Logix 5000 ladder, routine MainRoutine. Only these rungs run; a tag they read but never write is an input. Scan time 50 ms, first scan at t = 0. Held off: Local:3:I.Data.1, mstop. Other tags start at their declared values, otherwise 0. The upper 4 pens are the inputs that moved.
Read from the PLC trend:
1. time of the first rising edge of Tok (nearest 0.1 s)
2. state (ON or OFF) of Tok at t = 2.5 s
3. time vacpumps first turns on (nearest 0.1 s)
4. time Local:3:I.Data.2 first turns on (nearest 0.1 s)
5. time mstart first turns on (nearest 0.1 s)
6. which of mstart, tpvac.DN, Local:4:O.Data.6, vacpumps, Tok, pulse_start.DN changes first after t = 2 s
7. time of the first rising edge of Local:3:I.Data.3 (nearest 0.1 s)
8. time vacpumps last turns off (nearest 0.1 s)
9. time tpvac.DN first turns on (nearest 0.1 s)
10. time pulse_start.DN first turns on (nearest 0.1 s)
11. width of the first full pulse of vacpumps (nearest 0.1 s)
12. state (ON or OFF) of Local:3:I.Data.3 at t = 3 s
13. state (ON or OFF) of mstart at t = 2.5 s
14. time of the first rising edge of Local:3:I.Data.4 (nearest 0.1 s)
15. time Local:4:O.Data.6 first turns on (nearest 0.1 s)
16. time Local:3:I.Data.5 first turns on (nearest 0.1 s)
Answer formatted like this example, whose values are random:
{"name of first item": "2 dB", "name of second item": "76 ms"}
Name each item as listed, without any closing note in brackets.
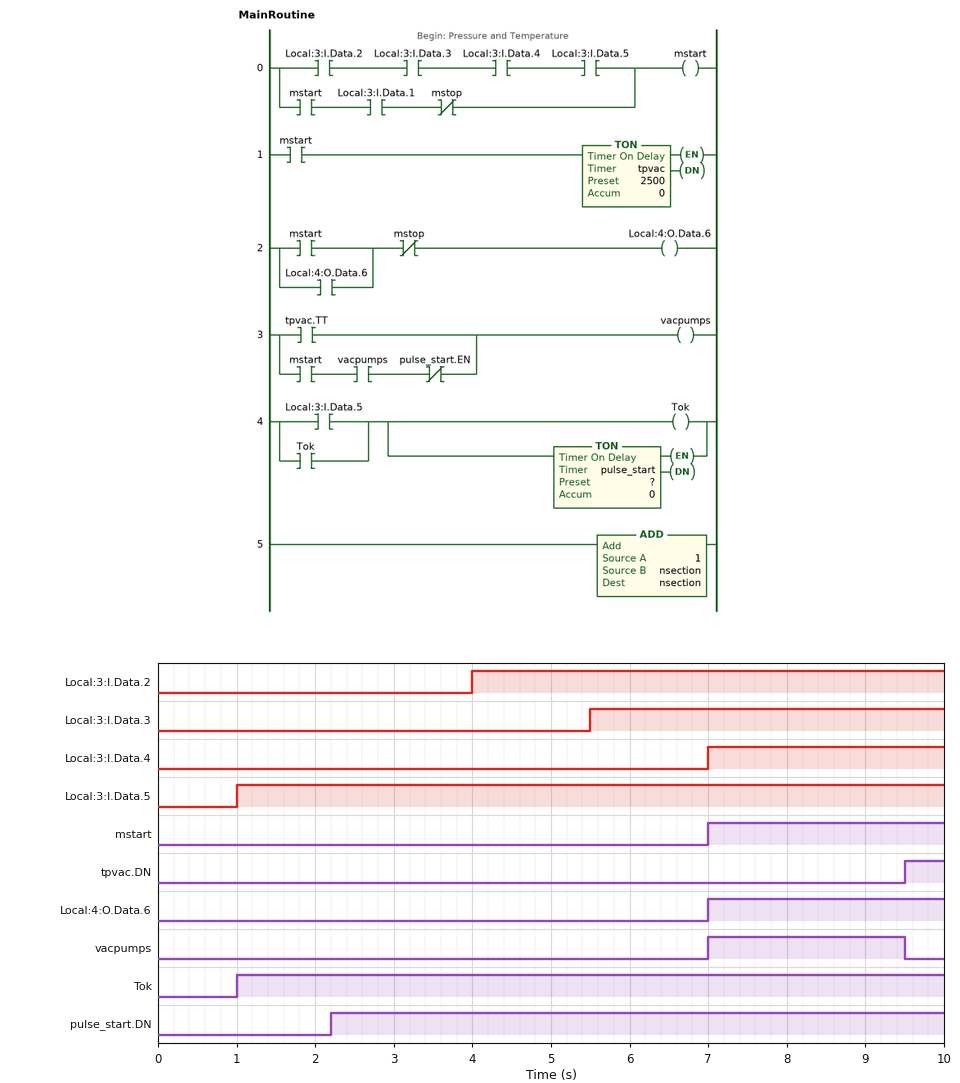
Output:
{"time of the first rising edge of Tok": "1.0 s", "state (ON or OFF) of Tok at t = 2.5 s": "ON", "time vacpumps first turns on": "7.0 s", "time Local:3:I.Data.2 first turns on": "4.0 s", "time mstart first turns on": "7.0 s", "which of mstart, tpvac.DN, Local:4:O.Data.6, vacpumps, Tok, pulse_start.DN changes first after t = 2 s": "pulse_start.DN", "time of the first rising edge of Local:3:I.Data.3": "5.5 s", "time vacpumps last turns off": "9.5 s", "time tpvac.DN first turns on": "9.5 s", "time pulse_start.DN first turns on": "2.2 s", "width of the first full pulse of vacpumps": "2.5 s", "state (ON or OFF) of Local:3:I.Data.3 at t = 3 s": "OFF", "state (ON or OFF) of mstart at t = 2.5 s": "OFF", "time of the first rising edge of Local:3:I.Data.4": "7.0 s", "time Local:4:O.Data.6 first turns on": "7.0 s", "time Local:3:I.Data.5 first turns on": "1.0 s"}
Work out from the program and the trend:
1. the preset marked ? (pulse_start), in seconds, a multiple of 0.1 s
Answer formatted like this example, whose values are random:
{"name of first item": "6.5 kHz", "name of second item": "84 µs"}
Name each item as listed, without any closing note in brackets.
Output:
{"the preset marked ? (pulse_start), in seconds, a multiple of 0.1 s": "1.2 s"}
